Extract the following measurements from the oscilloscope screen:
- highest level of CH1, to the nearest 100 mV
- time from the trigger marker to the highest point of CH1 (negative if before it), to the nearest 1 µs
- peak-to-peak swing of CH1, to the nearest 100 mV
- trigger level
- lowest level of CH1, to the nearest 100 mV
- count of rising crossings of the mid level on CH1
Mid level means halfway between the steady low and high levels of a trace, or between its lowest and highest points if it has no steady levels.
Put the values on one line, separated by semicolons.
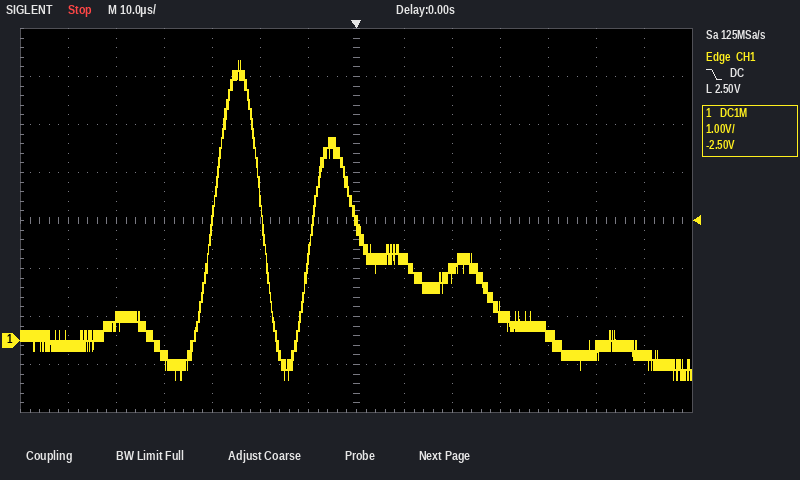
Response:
5.8 V; -24 µs; 6.6 V; 2.50 V; -800 mV; 2
